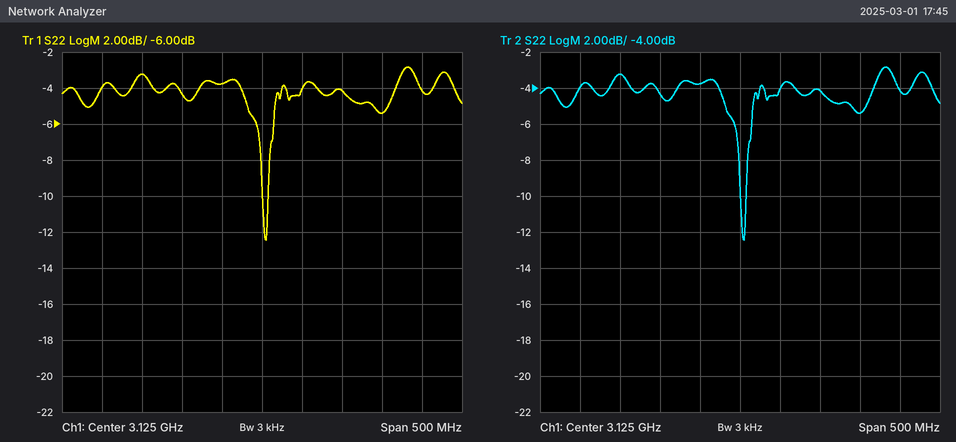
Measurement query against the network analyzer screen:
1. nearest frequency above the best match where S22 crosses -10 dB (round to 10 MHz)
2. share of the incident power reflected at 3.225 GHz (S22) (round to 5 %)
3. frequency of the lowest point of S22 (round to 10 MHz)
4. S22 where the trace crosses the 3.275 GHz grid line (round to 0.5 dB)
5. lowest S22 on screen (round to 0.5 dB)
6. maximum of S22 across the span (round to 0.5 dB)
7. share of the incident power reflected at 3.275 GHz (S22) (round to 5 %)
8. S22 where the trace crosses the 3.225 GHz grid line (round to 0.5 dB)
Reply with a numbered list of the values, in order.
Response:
1. 3.13 GHz
2. 40 %
3. 3.13 GHz
4. -5.5 dB
5. -12.5 dB
6. -3.0 dB
7. 30 %
8. -4.0 dB
